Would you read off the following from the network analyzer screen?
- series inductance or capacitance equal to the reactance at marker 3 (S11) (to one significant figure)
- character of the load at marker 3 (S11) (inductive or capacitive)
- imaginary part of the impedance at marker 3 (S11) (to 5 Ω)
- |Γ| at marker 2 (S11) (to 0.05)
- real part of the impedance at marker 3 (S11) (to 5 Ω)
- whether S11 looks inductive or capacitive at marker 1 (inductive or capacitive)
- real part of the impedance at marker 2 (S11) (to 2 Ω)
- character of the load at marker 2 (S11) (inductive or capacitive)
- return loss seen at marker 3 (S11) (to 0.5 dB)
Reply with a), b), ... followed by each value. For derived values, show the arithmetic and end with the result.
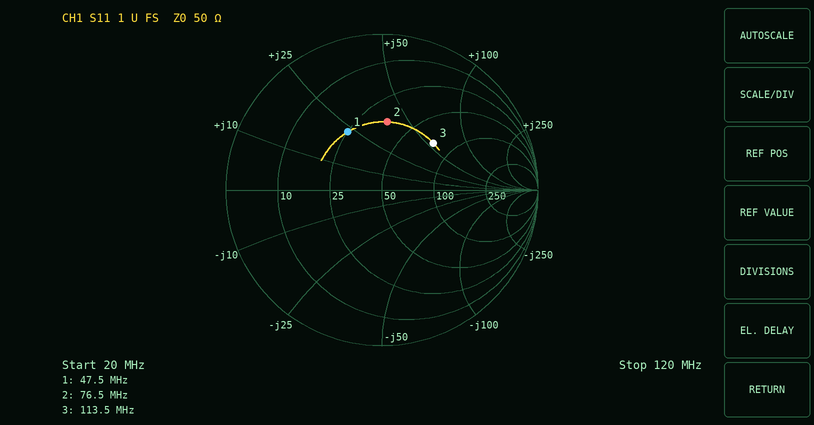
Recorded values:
a) L = 55 Ω/(2π × 113.5 MHz) ≈ 77.1 nH, so 80 nH to one significant figure
b) inductive
c) +55 Ω
d) 0.45
e) 75 Ω
f) inductive
g) 36 Ω
h) inductive
i) 7.0 dB
